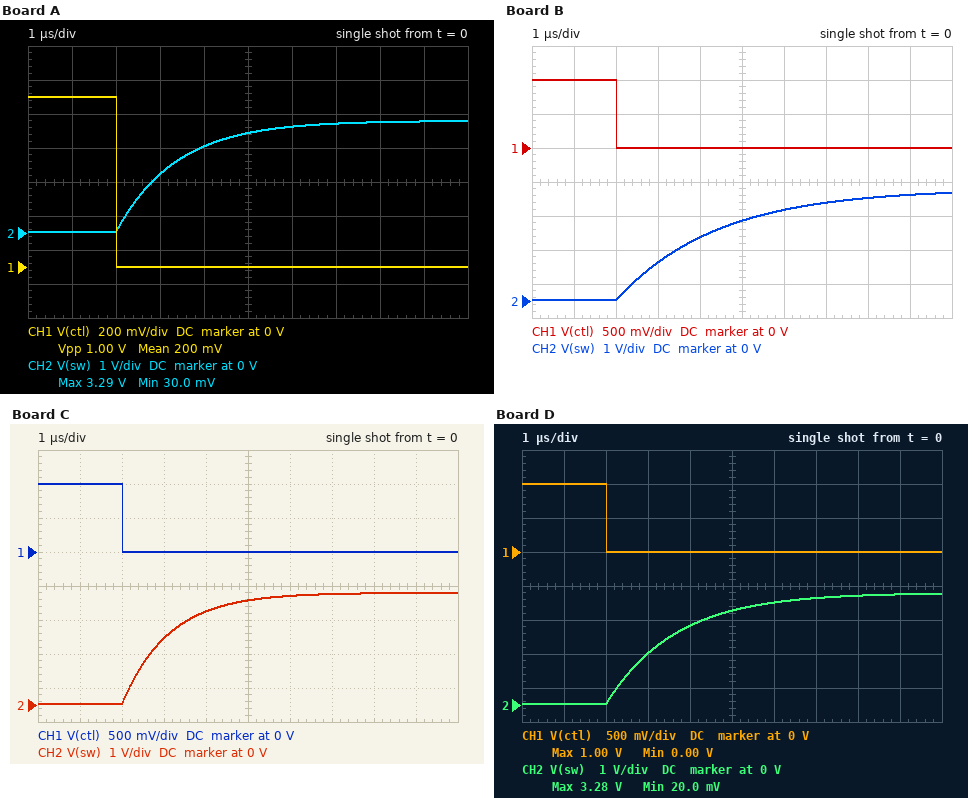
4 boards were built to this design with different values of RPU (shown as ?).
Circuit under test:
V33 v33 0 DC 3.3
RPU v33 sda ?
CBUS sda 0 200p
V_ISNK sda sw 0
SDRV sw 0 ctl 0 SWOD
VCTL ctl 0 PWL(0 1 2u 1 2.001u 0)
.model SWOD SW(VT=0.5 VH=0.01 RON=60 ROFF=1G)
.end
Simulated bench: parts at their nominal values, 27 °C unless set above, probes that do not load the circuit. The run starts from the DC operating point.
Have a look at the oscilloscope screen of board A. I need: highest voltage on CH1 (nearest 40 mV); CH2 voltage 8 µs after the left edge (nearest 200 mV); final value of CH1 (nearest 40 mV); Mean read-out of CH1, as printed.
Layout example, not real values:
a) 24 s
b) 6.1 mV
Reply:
a) 1.00 V
b) 3.2 V
c) 0 V
d) 200 mV
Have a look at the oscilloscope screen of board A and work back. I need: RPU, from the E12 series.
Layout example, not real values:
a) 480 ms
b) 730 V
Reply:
a) 6.8 kΩ
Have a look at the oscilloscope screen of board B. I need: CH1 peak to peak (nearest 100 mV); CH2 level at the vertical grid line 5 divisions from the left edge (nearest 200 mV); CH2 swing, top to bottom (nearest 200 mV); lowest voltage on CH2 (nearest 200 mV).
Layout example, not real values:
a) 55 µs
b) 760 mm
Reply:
a) 1.0 V
b) 2.4 V
c) 3.2 V
d) 0 V
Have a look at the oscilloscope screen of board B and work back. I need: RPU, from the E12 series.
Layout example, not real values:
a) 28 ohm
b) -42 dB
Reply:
a) 12 kΩ
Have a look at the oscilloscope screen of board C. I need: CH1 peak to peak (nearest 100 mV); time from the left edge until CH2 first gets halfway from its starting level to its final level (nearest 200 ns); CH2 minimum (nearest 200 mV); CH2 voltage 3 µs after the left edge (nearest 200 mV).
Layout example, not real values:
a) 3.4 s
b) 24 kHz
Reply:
a) 1.0 V
b) 2.8 µs
c) 0 V
d) 2.0 V
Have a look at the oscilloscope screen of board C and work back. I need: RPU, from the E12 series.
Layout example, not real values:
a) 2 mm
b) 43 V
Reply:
a) 5.6 kΩ
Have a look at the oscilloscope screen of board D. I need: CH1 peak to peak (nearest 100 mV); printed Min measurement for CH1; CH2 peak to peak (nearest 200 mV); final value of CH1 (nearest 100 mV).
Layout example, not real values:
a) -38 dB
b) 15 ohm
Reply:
a) 1.0 V
b) 0.00 V
c) 3.2 V
d) 0 V
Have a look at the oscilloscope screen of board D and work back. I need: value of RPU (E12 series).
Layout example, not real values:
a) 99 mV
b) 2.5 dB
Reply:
a) 8.2 kΩ
